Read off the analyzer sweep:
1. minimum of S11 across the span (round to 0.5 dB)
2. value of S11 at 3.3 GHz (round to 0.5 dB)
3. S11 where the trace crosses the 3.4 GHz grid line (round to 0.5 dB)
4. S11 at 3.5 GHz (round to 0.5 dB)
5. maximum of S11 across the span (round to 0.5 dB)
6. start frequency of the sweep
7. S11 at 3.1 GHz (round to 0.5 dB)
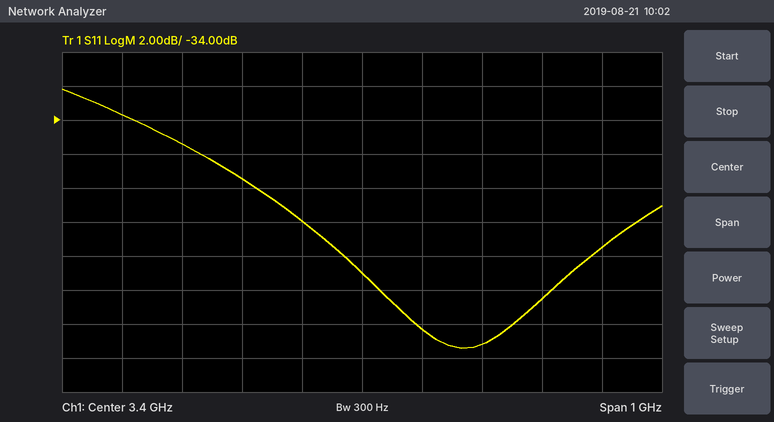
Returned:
-47.5 dB
-40.0 dB
-43.0 dB
-46.5 dB
-32.0 dB
2.9 GHz
-35.5 dB
